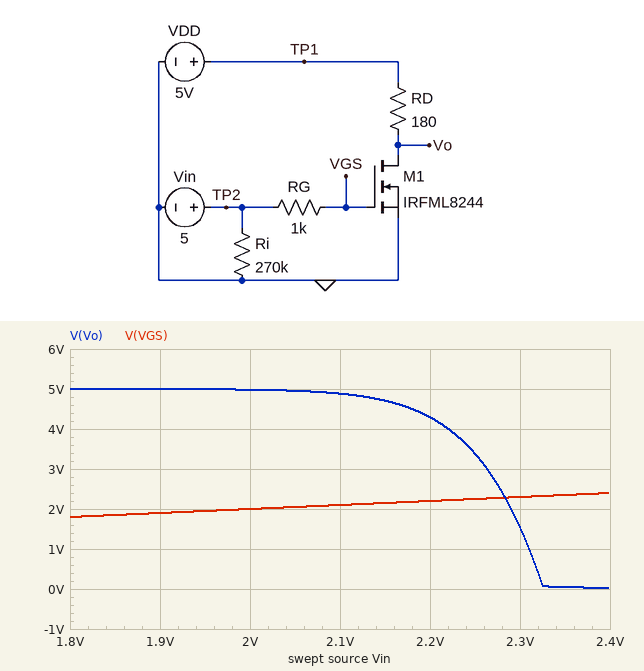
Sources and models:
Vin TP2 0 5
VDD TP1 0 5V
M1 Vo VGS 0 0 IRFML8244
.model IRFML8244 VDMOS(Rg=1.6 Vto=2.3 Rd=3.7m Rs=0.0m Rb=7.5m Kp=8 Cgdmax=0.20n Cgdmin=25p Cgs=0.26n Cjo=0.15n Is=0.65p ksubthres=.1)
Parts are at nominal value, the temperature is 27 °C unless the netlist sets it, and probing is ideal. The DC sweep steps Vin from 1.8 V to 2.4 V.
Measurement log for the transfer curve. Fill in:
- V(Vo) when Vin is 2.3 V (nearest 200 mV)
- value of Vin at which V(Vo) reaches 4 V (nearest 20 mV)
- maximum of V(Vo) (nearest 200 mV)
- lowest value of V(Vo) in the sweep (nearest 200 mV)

1.6 V
2.22 V
5.0 V
0 V
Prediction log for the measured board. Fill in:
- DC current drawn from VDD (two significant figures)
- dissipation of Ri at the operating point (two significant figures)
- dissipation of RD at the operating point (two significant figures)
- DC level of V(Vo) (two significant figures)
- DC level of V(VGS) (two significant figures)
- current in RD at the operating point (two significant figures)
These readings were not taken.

28 mA
93 µW
140 mW
1.4 mV
5.0 V
28 mA
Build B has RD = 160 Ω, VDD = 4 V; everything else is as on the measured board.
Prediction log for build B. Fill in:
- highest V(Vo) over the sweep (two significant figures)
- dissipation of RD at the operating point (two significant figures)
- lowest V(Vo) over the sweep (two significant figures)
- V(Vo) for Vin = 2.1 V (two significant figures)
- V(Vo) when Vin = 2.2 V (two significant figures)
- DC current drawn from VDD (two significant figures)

4.0 V
100 mW
26 mV
3.9 V
3.4 V
25 mA
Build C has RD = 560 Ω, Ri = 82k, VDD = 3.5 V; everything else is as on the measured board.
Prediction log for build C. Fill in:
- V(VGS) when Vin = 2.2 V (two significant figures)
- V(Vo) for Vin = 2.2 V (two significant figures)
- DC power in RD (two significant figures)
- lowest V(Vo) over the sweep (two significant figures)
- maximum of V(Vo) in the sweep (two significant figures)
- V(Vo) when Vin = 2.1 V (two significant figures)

2.2 V
1.3 V
22 mW
6.1 mV
3.5 V
3.1 V
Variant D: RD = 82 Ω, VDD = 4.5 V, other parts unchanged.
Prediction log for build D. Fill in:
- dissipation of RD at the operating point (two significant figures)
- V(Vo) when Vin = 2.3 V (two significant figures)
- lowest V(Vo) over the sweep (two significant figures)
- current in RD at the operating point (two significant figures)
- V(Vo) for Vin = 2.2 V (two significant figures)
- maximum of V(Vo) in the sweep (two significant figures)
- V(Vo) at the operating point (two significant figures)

250 mW
2.9 V
70 mV
55 mA
4.2 V
4.5 V
2.7 mV
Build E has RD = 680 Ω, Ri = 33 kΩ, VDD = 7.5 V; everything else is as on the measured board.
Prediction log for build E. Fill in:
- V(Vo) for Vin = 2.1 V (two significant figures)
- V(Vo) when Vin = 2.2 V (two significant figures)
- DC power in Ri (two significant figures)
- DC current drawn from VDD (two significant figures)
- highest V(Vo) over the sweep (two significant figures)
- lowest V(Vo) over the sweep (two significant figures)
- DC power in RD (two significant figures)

7.1 V
4.8 V
760 µW
11 mA
7.5 V
11 mV
83 mW
